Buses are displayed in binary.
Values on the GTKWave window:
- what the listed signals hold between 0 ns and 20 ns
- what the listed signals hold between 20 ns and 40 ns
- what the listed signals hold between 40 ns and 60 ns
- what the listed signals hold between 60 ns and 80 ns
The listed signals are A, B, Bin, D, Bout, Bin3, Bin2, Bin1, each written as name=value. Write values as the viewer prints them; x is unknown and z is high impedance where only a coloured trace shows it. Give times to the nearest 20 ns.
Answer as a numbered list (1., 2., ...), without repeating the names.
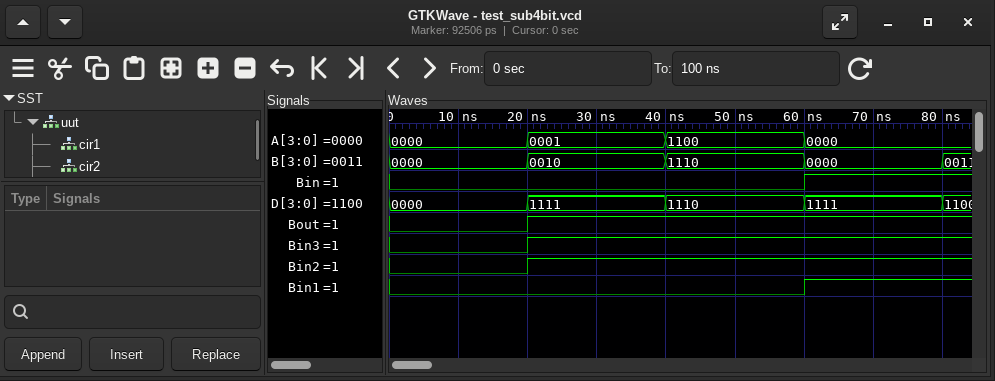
1. A=0000, B=0000, Bin=0, D=0000, Bout=0, Bin3=0, Bin2=0, Bin1=0
2. A=0001, B=0010, Bin=0, D=1111, Bout=1, Bin3=1, Bin2=1, Bin1=0
3. A=1100, B=1110, Bin=0, D=1110, Bout=1, Bin3=1, Bin2=1, Bin1=0
4. A=0000, B=0000, Bin=1, D=1111, Bout=1, Bin3=1, Bin2=1, Bin1=1
